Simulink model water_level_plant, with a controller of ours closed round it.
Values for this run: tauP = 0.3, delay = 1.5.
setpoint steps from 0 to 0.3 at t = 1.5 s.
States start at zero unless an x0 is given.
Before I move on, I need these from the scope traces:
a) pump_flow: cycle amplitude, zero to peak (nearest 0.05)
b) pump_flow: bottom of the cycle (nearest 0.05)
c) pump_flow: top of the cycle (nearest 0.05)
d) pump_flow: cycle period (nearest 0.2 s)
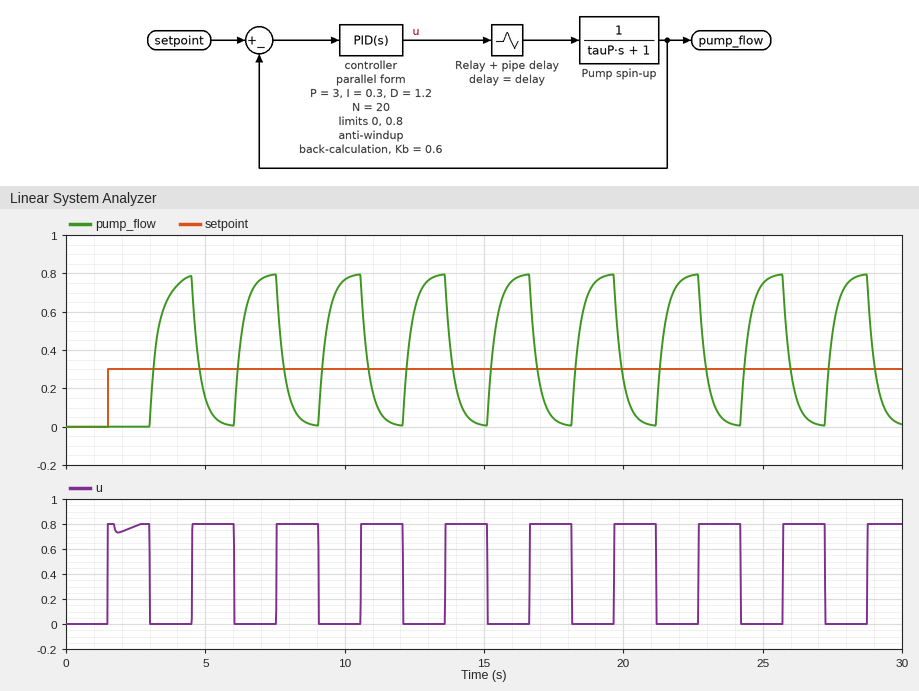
0.40
0.00
0.80
3.0 s
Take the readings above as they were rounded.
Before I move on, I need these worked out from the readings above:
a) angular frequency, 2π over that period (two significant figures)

2.1 rad/s
